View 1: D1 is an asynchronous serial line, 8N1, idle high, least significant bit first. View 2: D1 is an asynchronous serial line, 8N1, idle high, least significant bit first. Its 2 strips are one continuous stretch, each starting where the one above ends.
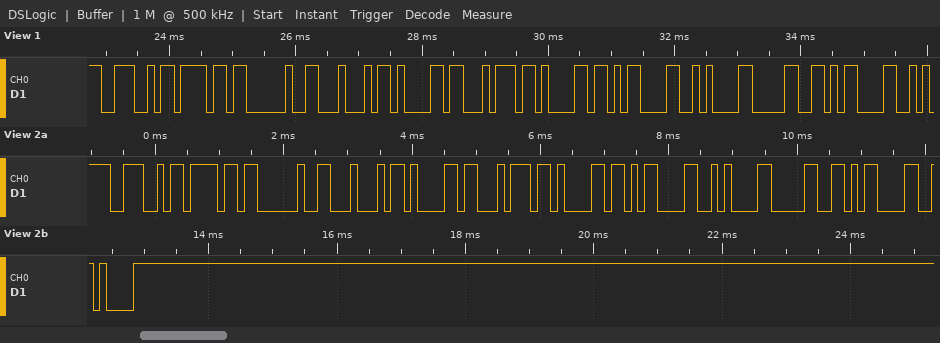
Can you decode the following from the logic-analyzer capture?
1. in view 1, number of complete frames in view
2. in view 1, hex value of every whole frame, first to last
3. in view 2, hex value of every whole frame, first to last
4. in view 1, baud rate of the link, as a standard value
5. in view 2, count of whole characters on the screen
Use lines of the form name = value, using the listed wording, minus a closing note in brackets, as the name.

in view 1, number of complete frames in view = 11
in view 1, hex value of every whole frame, first to last = 4E 6F 20 44 61 74 61 0D 0A 30 0D
in view 2, hex value of every whole frame, first to last = 4E 6F 20 44 61 74 61 0D 0A 30 0D 0A
in view 1, baud rate of the link, as a standard value = 9600 baud
in view 2, count of whole characters on the screen = 12
